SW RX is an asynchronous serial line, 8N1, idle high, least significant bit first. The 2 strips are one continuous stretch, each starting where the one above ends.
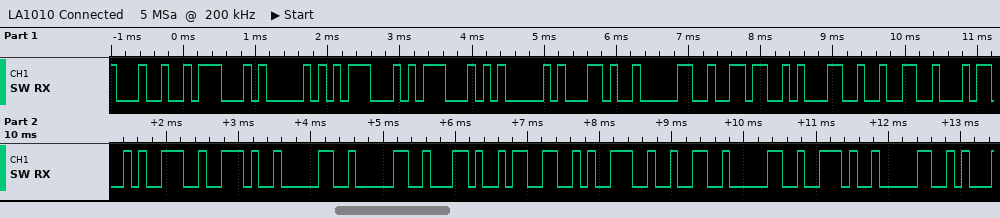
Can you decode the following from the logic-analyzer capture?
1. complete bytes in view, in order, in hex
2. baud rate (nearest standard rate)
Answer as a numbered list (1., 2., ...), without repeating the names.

1. 24 47 50 47 47 41 2C 30 36 31 32 34 39 2E 30 30 2C 33 39 32 30 2E 30
2. 9600 baud
